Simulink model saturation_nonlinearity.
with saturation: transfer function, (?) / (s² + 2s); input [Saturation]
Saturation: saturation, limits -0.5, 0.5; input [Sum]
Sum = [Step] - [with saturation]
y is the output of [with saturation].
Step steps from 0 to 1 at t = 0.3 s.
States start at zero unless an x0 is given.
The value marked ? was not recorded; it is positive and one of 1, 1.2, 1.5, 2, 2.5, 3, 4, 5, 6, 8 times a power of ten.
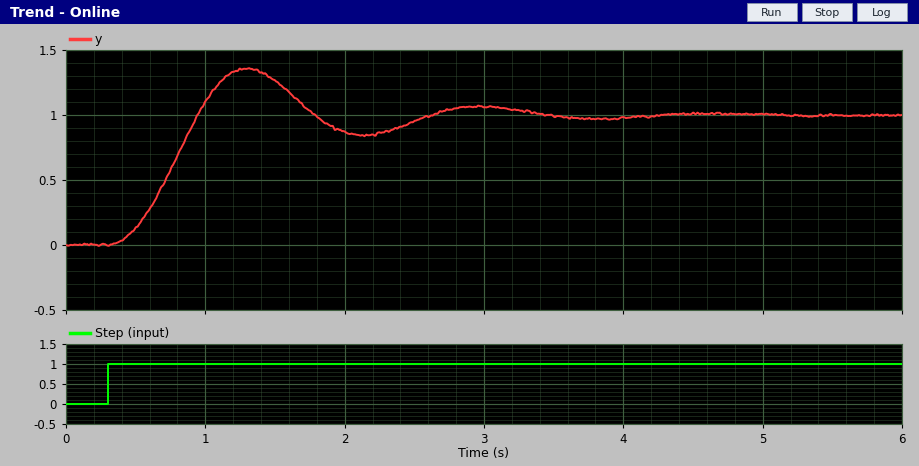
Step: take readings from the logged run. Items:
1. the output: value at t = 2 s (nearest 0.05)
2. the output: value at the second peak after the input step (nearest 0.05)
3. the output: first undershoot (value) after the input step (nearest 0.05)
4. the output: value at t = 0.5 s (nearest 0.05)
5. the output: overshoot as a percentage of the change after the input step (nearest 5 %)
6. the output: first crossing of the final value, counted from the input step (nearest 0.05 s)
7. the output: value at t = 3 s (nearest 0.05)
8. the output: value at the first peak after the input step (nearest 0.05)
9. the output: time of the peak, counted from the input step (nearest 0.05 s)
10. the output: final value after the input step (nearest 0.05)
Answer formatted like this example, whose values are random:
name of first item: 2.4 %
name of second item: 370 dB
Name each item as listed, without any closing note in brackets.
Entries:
the output: value at t = 2 s: 0.85
the output: value at the second peak after the input step: 1.05
the output: first undershoot (value) after the input step: 0.85
the output: value at t = 0.5 s: 0.15
the output: overshoot as a percentage of the change after the input step: 35 %
the output: first crossing of the final value, counted from the input step: 0.65 s
the output: value at t = 3 s: 1.05
the output: value at the first peak after the input step: 1.35
the output: time of the peak, counted from the input step: 1.00 s
the output: final value after the input step: 1.00
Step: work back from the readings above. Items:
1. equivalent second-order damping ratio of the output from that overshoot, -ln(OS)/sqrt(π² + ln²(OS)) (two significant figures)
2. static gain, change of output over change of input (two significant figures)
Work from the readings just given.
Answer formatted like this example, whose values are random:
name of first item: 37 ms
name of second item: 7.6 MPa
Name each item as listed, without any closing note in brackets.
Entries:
equivalent second-order damping ratio of the output from that overshoot, -ln(OS)/sqrt(π² + ln²(OS)): 0.32
static gain, change of output over change of input: 1.0
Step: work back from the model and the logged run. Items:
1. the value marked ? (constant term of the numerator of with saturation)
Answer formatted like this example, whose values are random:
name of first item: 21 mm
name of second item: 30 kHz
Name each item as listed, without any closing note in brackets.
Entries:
the value marked ?: 15
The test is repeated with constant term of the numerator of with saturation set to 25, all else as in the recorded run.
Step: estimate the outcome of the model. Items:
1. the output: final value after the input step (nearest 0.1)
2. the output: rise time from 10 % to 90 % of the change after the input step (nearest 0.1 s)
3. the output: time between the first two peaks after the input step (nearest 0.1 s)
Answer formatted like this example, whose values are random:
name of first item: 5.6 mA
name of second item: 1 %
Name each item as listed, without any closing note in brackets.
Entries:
the output: final value after the input step: 1.0
the output: rise time from 10 % to 90 % of the change after the input step: 0.3 s
the output: time between the first two peaks after the input step: 1.3 s
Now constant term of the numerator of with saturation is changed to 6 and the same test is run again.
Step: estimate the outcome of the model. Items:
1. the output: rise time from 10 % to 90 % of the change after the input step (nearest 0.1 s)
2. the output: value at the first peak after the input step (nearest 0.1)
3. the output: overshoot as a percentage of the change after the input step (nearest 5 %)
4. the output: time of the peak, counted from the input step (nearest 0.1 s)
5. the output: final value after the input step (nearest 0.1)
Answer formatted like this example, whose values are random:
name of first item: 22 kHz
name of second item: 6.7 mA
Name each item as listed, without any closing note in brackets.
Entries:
the output: rise time from 10 % to 90 % of the change after the input step: 0.8 s
the output: value at the first peak after the input step: 1.2
the output: overshoot as a percentage of the change after the input step: 20 %
the output: time of the peak, counted from the input step: 1.7 s
the output: final value after the input step: 1.0
